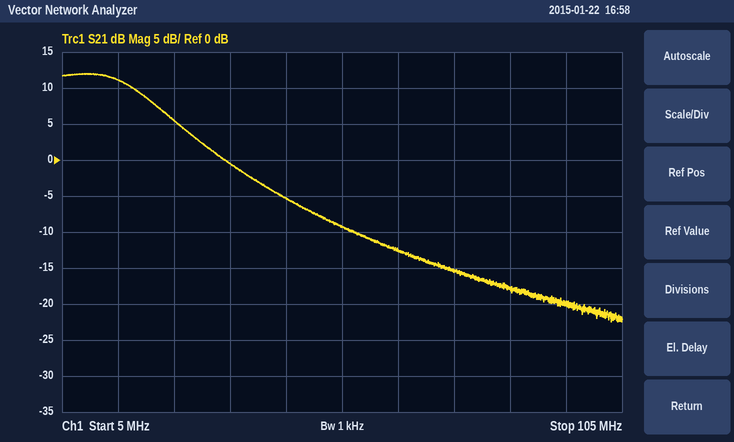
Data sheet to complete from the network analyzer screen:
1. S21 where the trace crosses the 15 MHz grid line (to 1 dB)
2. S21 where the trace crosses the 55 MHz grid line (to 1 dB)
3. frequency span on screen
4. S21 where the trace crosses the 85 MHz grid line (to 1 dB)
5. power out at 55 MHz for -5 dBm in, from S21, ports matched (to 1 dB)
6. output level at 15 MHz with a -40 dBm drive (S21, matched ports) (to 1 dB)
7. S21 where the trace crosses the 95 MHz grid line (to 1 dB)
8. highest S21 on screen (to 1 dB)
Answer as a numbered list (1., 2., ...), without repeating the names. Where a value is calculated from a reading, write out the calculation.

1. 11 dB
2. -9 dB
3. 100 MHz
4. -18 dB
5. -5 dBm + (-9 dB) = -14 dBm
6. -40 dBm + (11 dB) = -29 dBm
7. -20 dB
8. 12 dB
